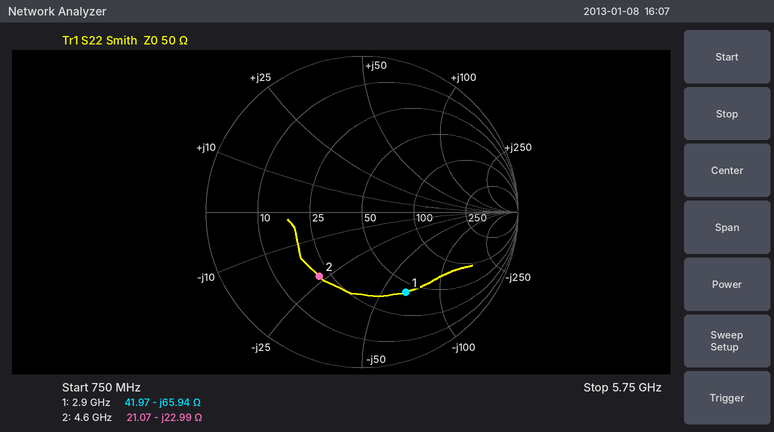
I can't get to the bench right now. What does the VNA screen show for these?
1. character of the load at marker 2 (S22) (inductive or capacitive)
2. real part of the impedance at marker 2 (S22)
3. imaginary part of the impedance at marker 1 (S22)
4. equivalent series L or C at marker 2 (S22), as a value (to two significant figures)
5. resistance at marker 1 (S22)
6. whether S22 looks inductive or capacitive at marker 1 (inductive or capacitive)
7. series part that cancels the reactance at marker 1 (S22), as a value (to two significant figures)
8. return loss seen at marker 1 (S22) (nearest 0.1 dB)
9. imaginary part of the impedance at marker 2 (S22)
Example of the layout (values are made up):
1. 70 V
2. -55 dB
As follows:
1. capacitive
2. 21.07 Ω
3. -65.94 Ω
4. 1.5 pF
5. 41.97 Ω
6. capacitive
7. 3.6 nH
8. 4.6 dB
9. -22.99 Ω
